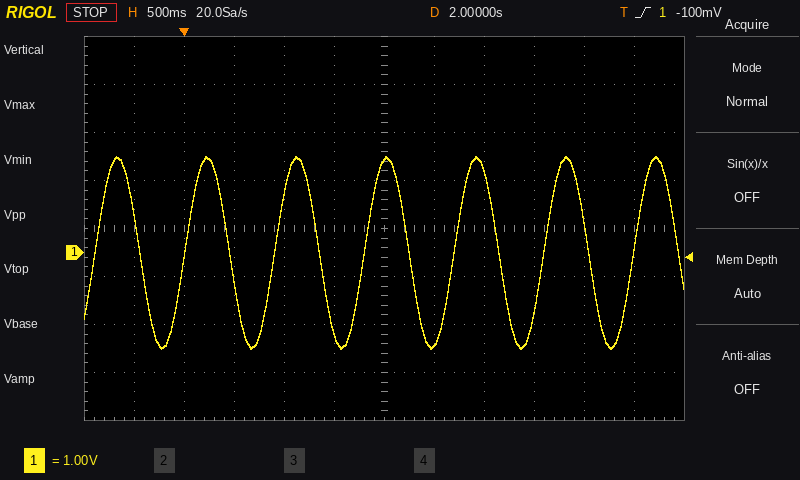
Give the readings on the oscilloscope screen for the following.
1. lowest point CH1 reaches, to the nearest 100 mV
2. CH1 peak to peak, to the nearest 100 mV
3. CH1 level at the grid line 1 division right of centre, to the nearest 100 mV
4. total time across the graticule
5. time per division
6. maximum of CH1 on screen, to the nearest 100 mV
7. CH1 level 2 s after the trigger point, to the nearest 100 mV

-2.0 V
4.0 V
-1.9 V
6 s
500 ms
2.0 V
1.9 V
